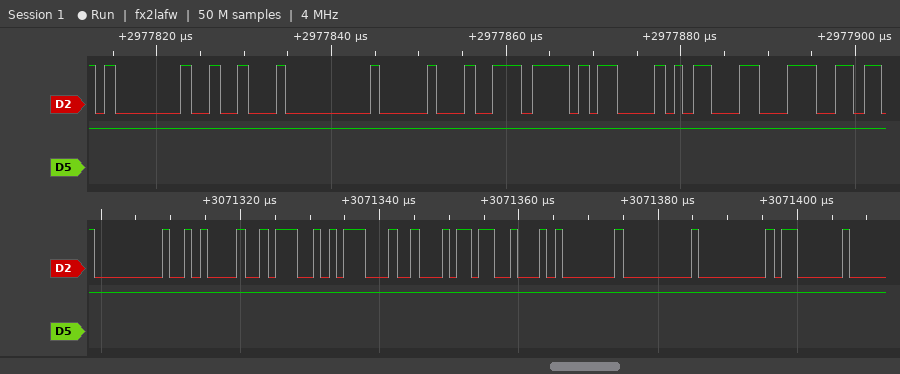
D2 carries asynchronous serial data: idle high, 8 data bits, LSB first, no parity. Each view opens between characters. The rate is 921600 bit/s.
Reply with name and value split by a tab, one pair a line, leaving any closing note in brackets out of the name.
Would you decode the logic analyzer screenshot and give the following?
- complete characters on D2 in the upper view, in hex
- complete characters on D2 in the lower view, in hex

complete characters on D2 in the upper view, in hex	01, 12, 00, 10, EE, 0D, 8D, 9C
complete characters on D2 in the lower view, in hex	00, 0A, 3A, 1D, A2, 13, 01, 00, 00, 03
